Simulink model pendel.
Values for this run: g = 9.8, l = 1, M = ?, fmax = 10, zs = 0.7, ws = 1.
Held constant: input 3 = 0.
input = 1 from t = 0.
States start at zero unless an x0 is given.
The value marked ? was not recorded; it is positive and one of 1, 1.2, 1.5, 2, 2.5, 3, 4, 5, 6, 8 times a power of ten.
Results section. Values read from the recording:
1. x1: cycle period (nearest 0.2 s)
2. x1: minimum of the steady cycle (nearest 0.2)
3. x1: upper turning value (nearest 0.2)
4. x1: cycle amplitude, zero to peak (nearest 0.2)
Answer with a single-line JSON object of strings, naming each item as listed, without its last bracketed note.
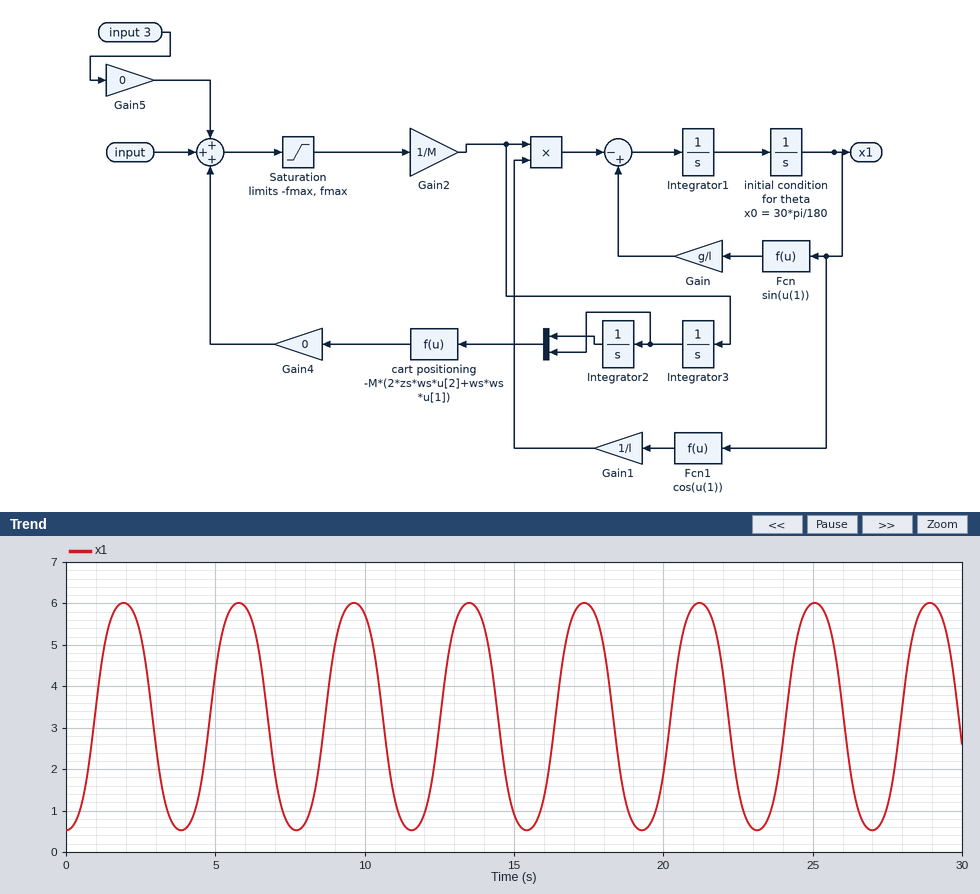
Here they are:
{"x1: cycle period": "3.8 s", "x1: minimum of the steady cycle": "0.6", "x1: upper turning value": "6.0", "x1: cycle amplitude, zero to peak": "2.8"}
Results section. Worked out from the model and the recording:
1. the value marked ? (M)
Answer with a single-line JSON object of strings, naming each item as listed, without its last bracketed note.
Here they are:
{"the value marked ?": "0.8"}
